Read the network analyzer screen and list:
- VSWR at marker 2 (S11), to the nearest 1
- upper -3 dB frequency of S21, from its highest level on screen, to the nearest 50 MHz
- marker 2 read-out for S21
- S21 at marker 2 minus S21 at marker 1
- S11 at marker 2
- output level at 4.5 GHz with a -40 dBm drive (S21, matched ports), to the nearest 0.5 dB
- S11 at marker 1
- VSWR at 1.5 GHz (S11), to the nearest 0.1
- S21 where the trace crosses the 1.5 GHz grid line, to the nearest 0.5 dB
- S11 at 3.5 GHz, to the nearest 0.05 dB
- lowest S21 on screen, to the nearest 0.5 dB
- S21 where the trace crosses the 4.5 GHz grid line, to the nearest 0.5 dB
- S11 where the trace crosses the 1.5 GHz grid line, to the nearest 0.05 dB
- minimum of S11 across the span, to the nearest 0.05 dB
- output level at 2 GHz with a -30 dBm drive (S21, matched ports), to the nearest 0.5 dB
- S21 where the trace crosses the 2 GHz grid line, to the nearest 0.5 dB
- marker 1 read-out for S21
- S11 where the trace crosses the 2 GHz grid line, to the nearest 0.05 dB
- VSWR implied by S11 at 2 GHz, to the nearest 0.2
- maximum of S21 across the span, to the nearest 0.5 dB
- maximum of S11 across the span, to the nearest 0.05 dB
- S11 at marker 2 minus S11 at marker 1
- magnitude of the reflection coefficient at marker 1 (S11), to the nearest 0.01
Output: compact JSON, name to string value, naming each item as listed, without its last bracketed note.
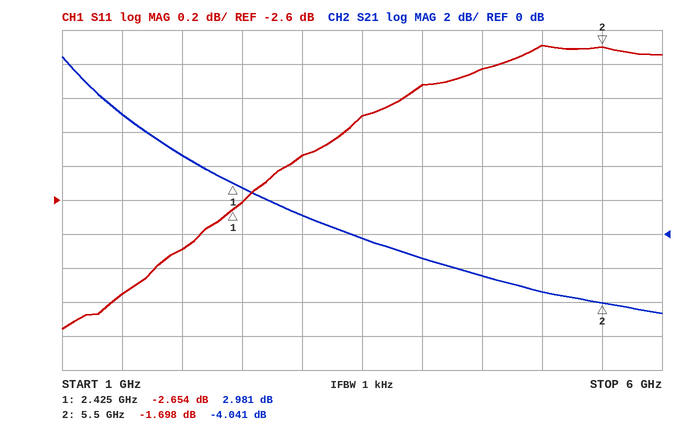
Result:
{"VSWR at marker 2 (S11), to the nearest 1": "10", "upper -3 dB frequency of S21, from its highest level on screen, to the nearest 50 MHz": "1.45 GHz", "marker 2 read-out for S21": "-4.041 dB", "S21 at marker 2 minus S21 at marker 1": "-7.022 dB", "S11 at marker 2": "-1.698 dB", "output level at 4.5 GHz with a -40 dBm drive (S21, matched ports), to the nearest 0.5 dB": "-42.5 dBm", "S11 at marker 1": "-2.654 dB", "VSWR at 1.5 GHz (S11), to the nearest 0.1": "5.6", "S21 where the trace crosses the 1.5 GHz grid line, to the nearest 0.5 dB": "7.0 dB", "S11 at 3.5 GHz, to the nearest 0.05 dB": "-2.10 dB", "lowest S21 on screen, to the nearest 0.5 dB": "-4.5 dB", "S21 where the trace crosses the 4.5 GHz grid line, to the nearest 0.5 dB": "-2.5 dB", "S11 where the trace crosses the 1.5 GHz grid line, to the nearest 0.05 dB": "-3.15 dB", "minimum of S11 across the span, to the nearest 0.05 dB": "-3.35 dB", "output level at 2 GHz with a -30 dBm drive (S21, matched ports), to the nearest 0.5 dB": "-25.5 dBm", "S21 where the trace crosses the 2 GHz grid line, to the nearest 0.5 dB": "4.5 dB", "marker 1 read-out for S21": "2.981 dB", "S11 where the trace crosses the 2 GHz grid line, to the nearest 0.05 dB": "-2.90 dB", "VSWR implied by S11 at 2 GHz, to the nearest 0.2": "6.0", "maximum of S21 across the span, to the nearest 0.5 dB": "10.5 dB", "maximum of S11 across the span, to the nearest 0.05 dB": "-1.70 dB", "S11 at marker 2 minus S11 at marker 1": "0.956 dB", "magnitude of the reflection coefficient at marker 1 (S11), to the nearest 0.01": "0.74"}
